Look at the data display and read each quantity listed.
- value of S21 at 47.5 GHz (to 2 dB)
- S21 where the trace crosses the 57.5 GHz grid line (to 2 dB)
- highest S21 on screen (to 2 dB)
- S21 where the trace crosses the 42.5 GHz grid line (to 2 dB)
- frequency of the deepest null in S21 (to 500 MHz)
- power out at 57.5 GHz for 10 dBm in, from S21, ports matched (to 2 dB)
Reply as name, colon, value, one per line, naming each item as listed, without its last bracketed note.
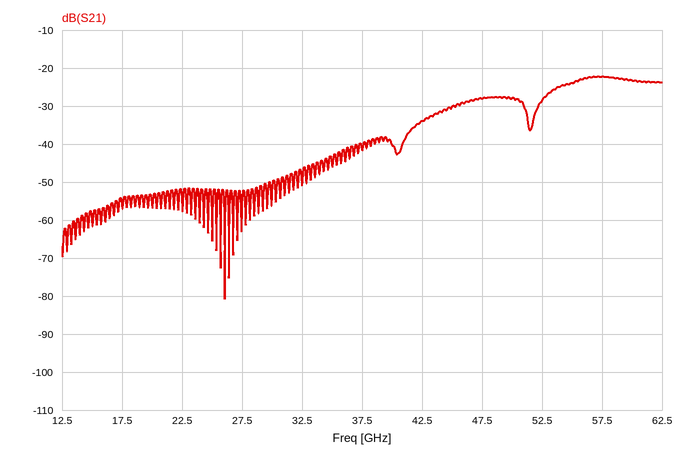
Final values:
value of S21 at 47.5 GHz: -28 dB
S21 where the trace crosses the 57.5 GHz grid line: -22 dB
highest S21 on screen: -22 dB
S21 where the trace crosses the 42.5 GHz grid line: -34 dB
frequency of the deepest null in S21: 26.0 GHz
power out at 57.5 GHz for 10 dBm in, from S21, ports matched: -12 dBm
